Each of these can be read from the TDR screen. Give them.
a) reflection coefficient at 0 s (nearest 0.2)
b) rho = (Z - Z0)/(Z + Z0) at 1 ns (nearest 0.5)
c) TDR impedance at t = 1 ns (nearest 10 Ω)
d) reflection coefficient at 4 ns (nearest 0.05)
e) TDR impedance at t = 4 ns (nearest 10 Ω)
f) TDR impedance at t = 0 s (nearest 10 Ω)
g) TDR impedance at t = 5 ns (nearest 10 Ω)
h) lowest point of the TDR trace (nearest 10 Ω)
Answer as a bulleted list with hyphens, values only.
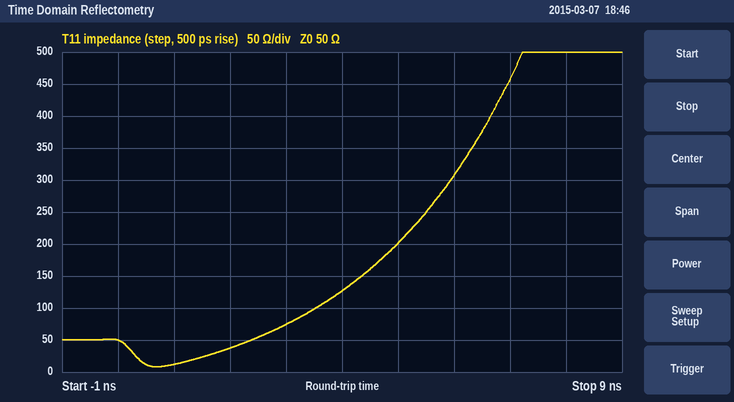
- 0.0
- -0.5
- 10 Ω
- +0.45
- 130 Ω
- 50 Ω
- 200 Ω
- 10 Ω
